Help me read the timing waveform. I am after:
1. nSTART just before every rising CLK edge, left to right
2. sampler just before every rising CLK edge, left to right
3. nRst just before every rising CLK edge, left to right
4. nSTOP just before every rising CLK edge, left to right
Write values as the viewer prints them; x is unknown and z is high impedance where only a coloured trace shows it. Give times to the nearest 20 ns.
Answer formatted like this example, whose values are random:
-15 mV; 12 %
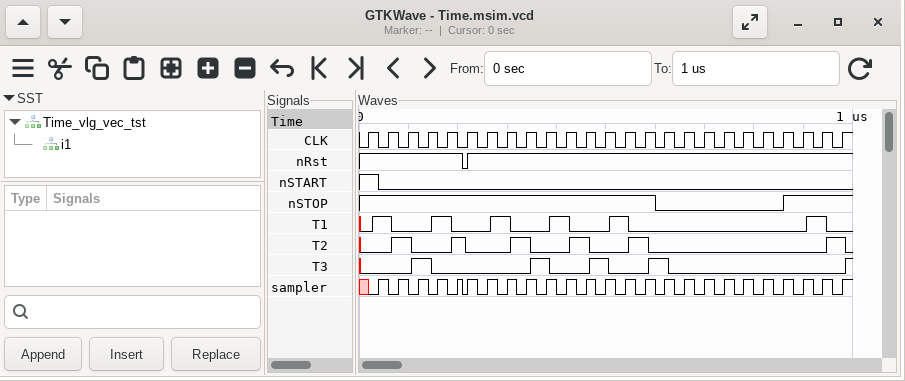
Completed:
1 0 0 0 0 0 0 0 0 0 0 0 0 0 0 0 0 0 0 0 0 0 0 0 0; x 1 1 1 1 0 0 0 0 0 0 0 0 0 0 0 0 0 0 0 0 0 0 0 0; 1 1 1 1 1 0 1 1 1 1 1 1 1 1 1 1 1 1 1 1 1 1 1 1 1; 1 1 1 1 1 1 1 1 1 1 1 1 1 1 1 0 0 0 0 0 0 0 1 1 1
